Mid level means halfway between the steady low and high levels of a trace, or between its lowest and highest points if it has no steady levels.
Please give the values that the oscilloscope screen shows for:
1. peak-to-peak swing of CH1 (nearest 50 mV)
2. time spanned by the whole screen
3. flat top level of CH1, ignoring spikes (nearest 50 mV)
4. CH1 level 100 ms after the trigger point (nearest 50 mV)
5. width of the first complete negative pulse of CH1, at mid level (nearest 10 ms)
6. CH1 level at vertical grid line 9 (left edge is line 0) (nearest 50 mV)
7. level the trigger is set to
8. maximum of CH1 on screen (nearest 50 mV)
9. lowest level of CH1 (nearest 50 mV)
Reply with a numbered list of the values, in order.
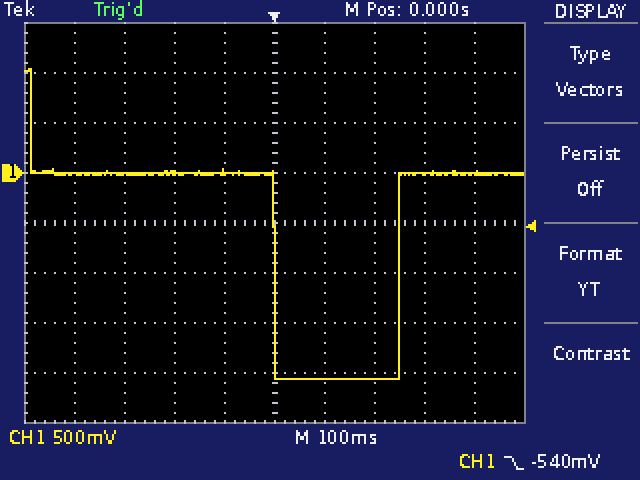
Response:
1. 3.10 V
2. 1 s
3. 0 mV
4. -2.05 V
5. 250 ms
6. 0 mV
7. -540 mV
8. 1.05 V
9. -2.05 V
